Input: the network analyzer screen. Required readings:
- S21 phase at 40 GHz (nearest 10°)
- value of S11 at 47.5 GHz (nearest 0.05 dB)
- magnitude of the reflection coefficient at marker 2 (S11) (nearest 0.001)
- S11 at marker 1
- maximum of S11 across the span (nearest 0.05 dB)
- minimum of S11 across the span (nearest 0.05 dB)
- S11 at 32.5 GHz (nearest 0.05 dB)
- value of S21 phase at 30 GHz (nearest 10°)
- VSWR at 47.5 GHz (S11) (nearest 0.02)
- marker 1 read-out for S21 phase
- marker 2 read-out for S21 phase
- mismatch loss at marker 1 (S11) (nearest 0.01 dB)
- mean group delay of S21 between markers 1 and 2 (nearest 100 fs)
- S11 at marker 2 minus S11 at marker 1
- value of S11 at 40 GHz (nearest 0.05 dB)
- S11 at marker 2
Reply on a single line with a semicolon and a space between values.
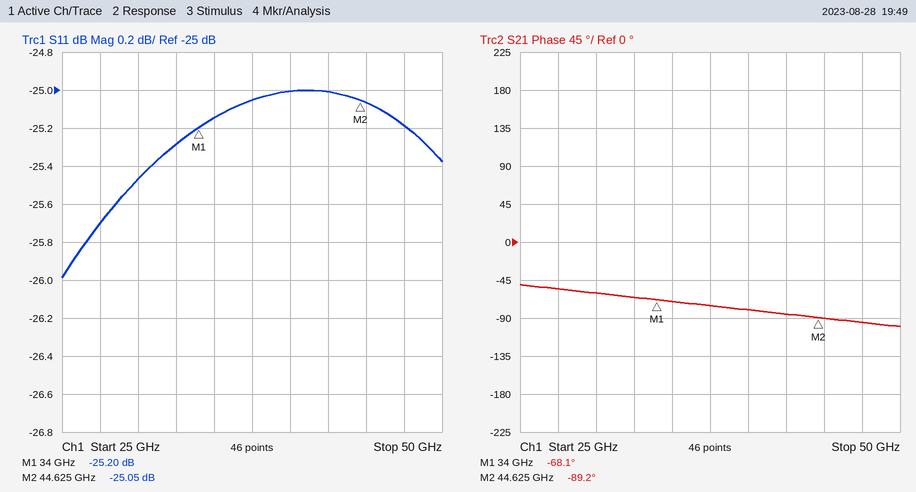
-80°; -25.20 dB; 0.056; -25.20 dB; -25.00 dB; -26.00 dB; -25.30 dB; -60°; 1.12; -68.1°; -89.2°; 0.01 dB; 5.5 ps; 0.15 dB; -25.00 dB; -25.05 dB
